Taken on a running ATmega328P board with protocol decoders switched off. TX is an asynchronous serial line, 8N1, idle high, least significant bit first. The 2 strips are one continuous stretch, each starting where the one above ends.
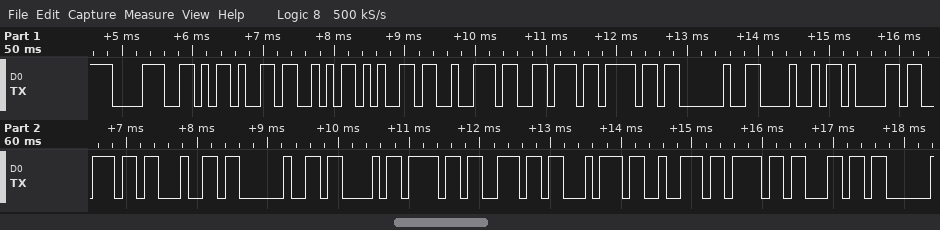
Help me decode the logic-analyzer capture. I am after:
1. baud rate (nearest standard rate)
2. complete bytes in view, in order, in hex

9600 baud
0x38 0x2D 0x53 0x65 0x72 0x76 0x6F 0x20 0x48 0x61 0x6E 0x64 0x20 0x43 0x6F 0x6E 0x74 0x72 0x6F 0x6C
